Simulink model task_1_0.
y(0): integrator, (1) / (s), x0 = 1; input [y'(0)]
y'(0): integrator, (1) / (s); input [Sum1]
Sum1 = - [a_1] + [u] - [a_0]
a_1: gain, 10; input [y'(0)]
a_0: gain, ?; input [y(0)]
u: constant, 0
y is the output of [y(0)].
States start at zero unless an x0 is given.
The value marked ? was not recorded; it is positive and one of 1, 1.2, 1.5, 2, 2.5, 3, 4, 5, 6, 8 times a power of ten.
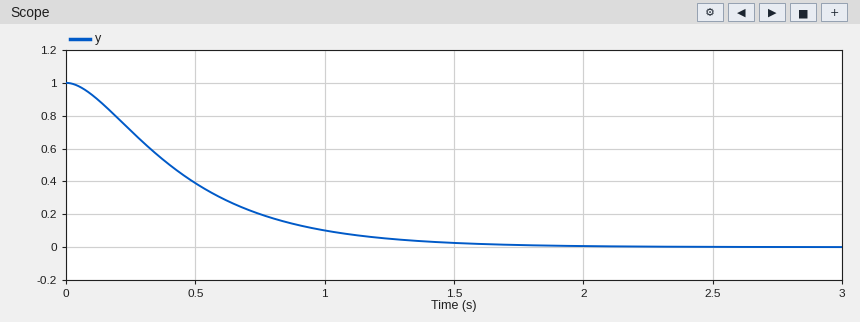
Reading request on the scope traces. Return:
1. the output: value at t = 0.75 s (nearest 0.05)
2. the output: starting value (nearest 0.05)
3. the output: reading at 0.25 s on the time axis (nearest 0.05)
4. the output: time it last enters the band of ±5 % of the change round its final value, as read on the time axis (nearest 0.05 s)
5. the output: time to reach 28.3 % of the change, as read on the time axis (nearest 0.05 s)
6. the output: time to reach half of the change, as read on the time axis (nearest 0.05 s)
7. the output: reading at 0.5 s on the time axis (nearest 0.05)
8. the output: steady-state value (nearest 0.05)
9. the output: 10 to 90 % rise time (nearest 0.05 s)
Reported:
0.20
1.00
0.70
1.25 s
0.25 s
0.40 s
0.40
0.00
0.90 s
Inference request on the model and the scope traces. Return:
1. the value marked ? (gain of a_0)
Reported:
20
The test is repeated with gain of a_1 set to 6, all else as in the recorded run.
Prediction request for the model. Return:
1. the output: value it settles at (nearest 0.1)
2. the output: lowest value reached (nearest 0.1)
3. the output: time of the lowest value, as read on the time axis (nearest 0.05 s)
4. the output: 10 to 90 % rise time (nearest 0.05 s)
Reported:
0.0
-0.1
0.95 s
0.45 s
